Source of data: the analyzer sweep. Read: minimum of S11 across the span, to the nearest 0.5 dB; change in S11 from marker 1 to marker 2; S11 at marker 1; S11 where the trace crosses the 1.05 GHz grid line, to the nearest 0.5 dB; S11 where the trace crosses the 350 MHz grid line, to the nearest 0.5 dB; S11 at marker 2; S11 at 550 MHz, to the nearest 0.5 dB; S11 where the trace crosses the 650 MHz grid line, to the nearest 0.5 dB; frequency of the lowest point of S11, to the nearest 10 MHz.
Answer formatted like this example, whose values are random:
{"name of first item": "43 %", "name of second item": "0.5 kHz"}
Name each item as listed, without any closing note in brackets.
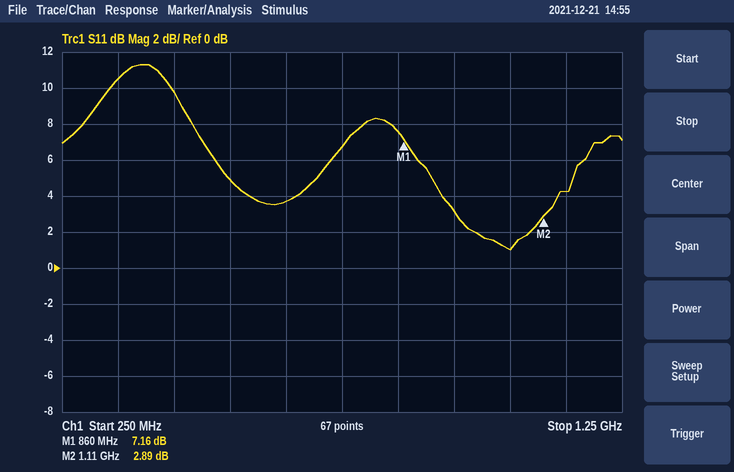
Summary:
{"minimum of S11 across the span, to the nearest 0.5 dB": "1.0 dB", "change in S11 from marker 1 to marker 2": "-4.27 dB", "S11 at marker 1": "7.16 dB", "S11 where the trace crosses the 1.05 GHz grid line, to the nearest 0.5 dB": "1.0 dB", "S11 where the trace crosses the 350 MHz grid line, to the nearest 0.5 dB": "10.5 dB", "S11 at marker 2": "2.89 dB", "S11 at 550 MHz, to the nearest 0.5 dB": "5.0 dB", "S11 where the trace crosses the 650 MHz grid line, to the nearest 0.5 dB": "3.5 dB", "frequency of the lowest point of S11, to the nearest 10 MHz": "1.05 GHz"}
